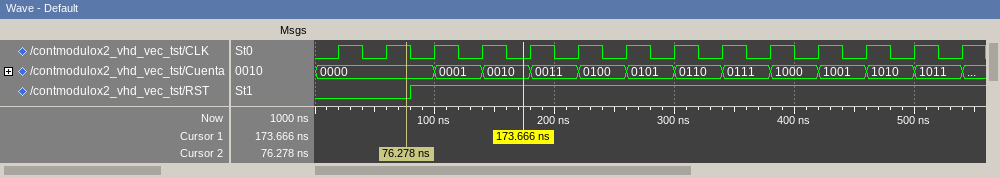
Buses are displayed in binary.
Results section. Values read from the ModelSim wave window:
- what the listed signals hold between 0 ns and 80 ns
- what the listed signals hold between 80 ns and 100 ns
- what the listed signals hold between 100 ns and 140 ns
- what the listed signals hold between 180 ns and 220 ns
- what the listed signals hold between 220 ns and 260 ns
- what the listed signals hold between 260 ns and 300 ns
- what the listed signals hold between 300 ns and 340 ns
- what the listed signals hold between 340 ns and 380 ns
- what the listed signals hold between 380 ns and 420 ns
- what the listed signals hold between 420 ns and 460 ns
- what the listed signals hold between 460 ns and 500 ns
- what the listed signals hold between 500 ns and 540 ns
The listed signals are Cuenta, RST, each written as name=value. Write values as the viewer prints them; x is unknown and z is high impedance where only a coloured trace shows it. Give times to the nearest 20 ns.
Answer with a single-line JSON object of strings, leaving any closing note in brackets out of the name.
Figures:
{"what the listed signals hold between 0 ns and 80 ns": "Cuenta=0000, RST=0", "what the listed signals hold between 80 ns and 100 ns": "Cuenta=0000, RST=1", "what the listed signals hold between 100 ns and 140 ns": "Cuenta=0001, RST=1", "what the listed signals hold between 180 ns and 220 ns": "Cuenta=0011, RST=1", "what the listed signals hold between 220 ns and 260 ns": "Cuenta=0100, RST=1", "what the listed signals hold between 260 ns and 300 ns": "Cuenta=0101, RST=1", "what the listed signals hold between 300 ns and 340 ns": "Cuenta=0110, RST=1", "what the listed signals hold between 340 ns and 380 ns": "Cuenta=0111, RST=1", "what the listed signals hold between 380 ns and 420 ns": "Cuenta=1000, RST=1", "what the listed signals hold between 420 ns and 460 ns": "Cuenta=1001, RST=1", "what the listed signals hold between 460 ns and 500 ns": "Cuenta=1010, RST=1", "what the listed signals hold between 500 ns and 540 ns": "Cuenta=1011, RST=1"}
